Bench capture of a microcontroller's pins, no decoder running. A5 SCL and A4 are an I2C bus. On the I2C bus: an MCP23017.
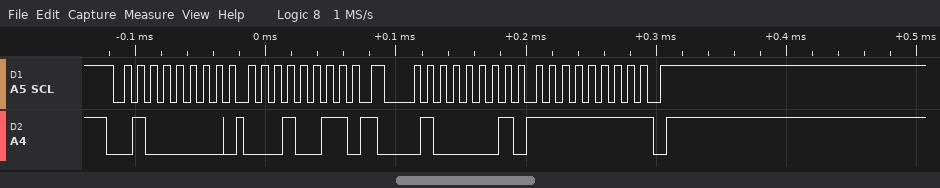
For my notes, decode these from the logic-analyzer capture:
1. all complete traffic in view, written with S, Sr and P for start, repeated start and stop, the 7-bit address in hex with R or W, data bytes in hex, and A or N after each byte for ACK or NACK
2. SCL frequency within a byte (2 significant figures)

S 20W A 13 A Sr 20R A FF N P
100 kHz
